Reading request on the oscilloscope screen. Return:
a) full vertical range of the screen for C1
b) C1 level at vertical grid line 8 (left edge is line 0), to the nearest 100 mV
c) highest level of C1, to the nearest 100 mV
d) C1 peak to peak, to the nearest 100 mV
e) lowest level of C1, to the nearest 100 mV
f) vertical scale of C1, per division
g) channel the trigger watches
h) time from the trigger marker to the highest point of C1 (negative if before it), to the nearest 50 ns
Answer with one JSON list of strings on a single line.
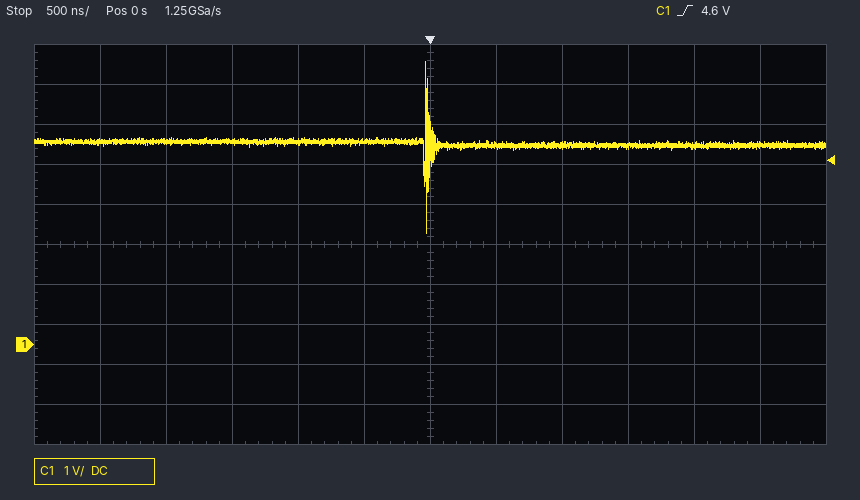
["10 V", "5.0 V", "7.1 V", "4.3 V", "2.8 V", "1 V", "C1", "-50 ns"]
